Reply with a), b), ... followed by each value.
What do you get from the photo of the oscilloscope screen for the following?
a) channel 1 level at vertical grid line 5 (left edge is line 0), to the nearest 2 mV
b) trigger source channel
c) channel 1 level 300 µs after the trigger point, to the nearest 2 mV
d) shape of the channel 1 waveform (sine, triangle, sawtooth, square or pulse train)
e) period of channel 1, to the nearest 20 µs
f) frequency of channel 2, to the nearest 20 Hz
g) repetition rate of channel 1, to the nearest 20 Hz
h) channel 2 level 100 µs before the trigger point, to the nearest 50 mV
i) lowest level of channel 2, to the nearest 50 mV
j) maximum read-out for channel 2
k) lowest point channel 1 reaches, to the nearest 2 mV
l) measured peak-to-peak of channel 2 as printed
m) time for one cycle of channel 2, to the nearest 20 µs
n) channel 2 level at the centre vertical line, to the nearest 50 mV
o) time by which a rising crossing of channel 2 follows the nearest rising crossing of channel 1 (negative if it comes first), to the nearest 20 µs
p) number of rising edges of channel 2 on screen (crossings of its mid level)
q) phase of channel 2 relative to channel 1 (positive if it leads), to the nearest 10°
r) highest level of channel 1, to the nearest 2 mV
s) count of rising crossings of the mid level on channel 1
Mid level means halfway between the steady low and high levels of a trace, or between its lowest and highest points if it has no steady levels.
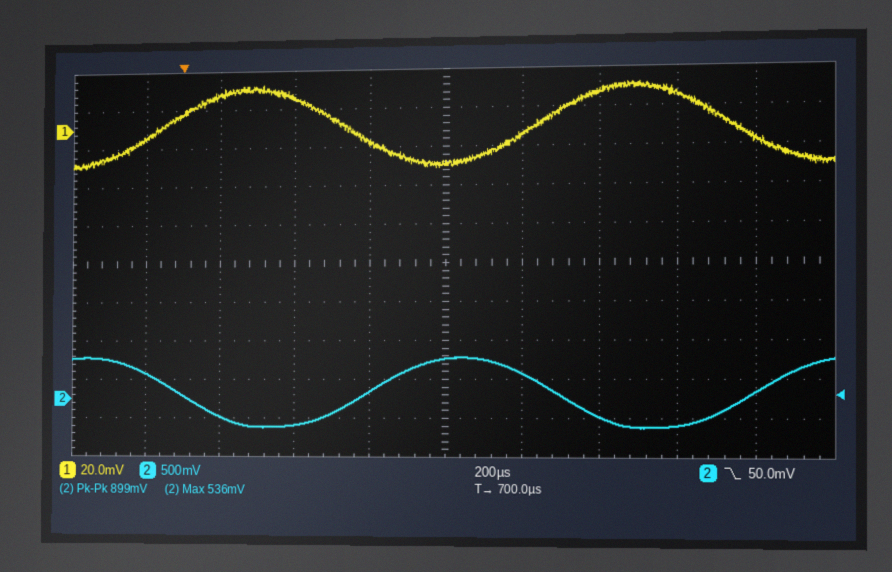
a) -18 mV
b) channel 2
c) 16 mV
d) sine
e) 1.00 ms
f) 1.00 kHz
g) 1.00 kHz
h) 350 mV
i) -350 mV
j) 536 mV
k) -20 mV
l) 899 mV
m) 1.00 ms
n) 500 mV
o) -440 µs
p) 2
q) +160°
r) 22 mV
s) 2
